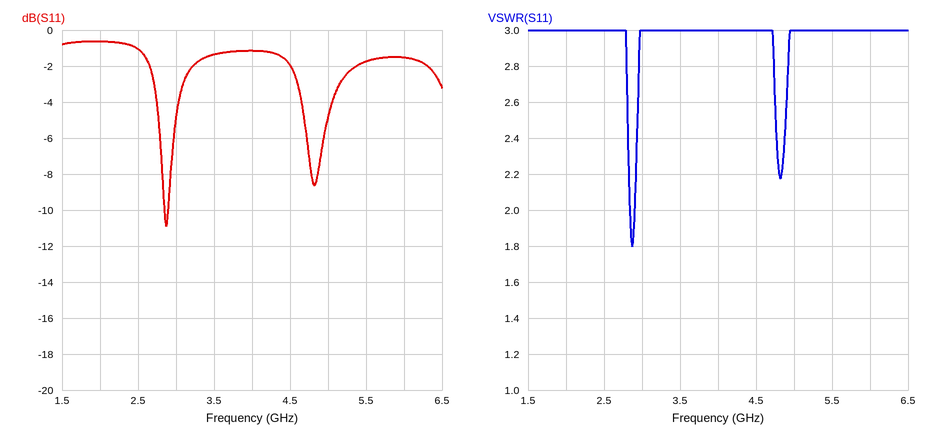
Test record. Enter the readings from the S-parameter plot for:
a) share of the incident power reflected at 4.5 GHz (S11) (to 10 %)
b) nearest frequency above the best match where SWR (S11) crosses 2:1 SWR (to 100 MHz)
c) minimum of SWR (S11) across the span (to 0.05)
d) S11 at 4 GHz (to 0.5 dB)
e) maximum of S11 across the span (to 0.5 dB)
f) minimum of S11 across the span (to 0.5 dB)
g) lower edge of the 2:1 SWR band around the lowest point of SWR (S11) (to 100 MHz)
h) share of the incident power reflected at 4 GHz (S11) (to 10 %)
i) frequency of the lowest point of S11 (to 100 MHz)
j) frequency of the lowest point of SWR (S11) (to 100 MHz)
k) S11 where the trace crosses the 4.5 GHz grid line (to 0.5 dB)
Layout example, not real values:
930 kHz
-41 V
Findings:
60 %
2.9 GHz
1.80
-1.0 dB
-0.5 dB
-11.0 dB
2.8 GHz
80 %
2.9 GHz
2.9 GHz
-2.0 dB
